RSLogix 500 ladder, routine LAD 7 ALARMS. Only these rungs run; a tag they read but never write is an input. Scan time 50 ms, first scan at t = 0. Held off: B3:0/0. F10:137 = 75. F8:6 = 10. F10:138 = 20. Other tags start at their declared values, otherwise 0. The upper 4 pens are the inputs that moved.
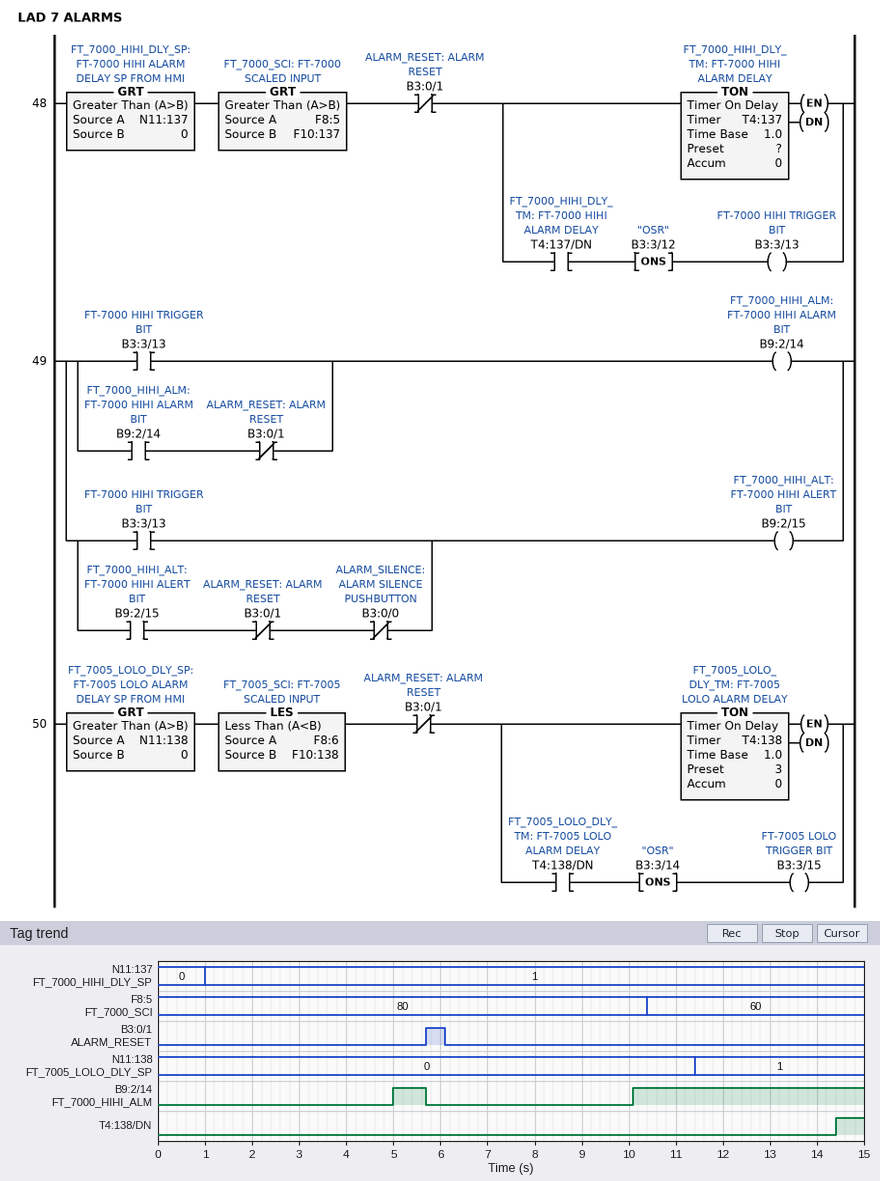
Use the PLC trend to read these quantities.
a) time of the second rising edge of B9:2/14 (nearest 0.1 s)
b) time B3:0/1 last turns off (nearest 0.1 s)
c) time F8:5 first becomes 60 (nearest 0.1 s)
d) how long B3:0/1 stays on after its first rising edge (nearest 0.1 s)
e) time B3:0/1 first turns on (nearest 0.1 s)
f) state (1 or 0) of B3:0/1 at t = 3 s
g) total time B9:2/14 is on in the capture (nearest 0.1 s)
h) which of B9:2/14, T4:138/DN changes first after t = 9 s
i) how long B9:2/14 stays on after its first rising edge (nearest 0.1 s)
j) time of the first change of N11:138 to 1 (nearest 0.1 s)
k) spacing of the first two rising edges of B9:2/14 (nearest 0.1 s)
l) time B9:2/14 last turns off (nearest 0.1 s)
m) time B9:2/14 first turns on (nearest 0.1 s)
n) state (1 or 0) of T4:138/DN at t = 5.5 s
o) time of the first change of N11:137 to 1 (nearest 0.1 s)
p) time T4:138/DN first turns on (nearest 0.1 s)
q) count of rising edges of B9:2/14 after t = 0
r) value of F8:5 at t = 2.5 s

10.1 s
6.1 s
10.4 s
0.4 s
5.7 s
0
5.6 s
B9:2/14
0.7 s
11.4 s
5.1 s
5.7 s
5.0 s
0
1.0 s
14.4 s
2
80
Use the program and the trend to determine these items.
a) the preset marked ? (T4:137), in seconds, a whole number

4 s
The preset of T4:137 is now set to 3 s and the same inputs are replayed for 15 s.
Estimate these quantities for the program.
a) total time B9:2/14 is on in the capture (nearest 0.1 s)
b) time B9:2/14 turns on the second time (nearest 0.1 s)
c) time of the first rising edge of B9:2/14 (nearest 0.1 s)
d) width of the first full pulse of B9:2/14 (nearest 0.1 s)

7.6 s
9.1 s
4.0 s
1.7 s
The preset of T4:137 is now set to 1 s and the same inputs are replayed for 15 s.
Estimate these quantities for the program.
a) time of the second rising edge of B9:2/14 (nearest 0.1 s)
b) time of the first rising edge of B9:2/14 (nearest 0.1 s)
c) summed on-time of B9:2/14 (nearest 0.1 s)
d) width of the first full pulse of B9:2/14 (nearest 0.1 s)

7.1 s
2.0 s
11.6 s
3.7 s
